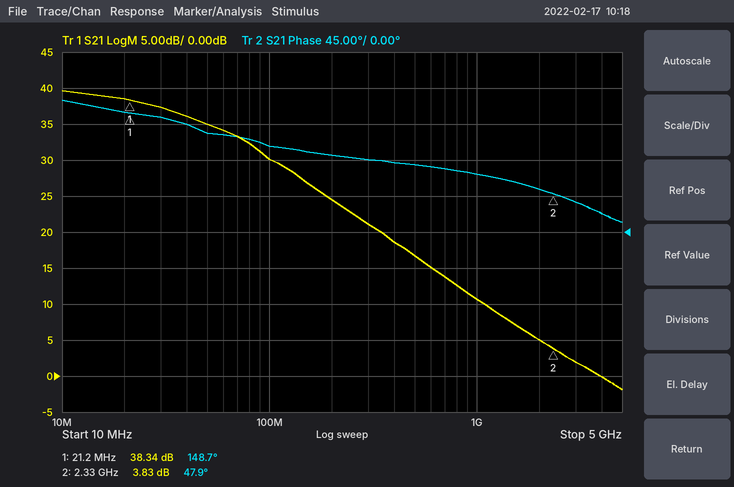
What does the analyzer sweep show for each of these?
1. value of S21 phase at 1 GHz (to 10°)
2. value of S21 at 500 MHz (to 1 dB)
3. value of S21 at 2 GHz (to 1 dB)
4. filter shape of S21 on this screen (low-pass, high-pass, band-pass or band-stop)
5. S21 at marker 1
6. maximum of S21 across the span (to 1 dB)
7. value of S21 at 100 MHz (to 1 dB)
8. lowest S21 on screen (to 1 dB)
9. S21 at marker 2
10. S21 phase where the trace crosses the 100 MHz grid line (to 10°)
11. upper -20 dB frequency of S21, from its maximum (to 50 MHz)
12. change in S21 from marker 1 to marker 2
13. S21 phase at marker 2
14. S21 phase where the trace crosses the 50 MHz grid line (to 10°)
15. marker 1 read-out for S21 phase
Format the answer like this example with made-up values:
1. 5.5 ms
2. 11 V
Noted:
1. 70°
2. 17 dB
3. 5 dB
4. low-pass
5. 38.34 dB
6. 40 dB
7. 30 dB
8. -2 dB
9. 3.83 dB
10. 110°
11. 350 MHz
12. -34.51 dB
13. 47.9°
14. 120°
15. 148.7°
